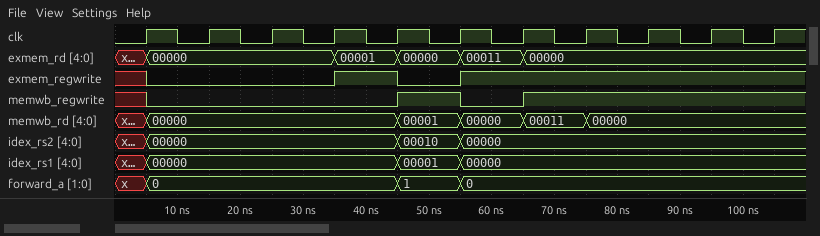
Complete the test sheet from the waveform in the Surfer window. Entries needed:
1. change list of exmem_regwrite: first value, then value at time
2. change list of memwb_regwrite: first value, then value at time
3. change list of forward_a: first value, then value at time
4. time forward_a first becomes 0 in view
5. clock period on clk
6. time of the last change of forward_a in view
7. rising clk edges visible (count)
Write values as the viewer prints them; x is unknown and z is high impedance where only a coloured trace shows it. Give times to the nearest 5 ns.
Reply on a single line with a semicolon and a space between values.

x, 0 at 5 ns, 1 at 35 ns, 0 at 45 ns, 1 at 55 ns; x, 0 at 5 ns, 1 at 45 ns, 0 at 55 ns, 1 at 65 ns; x, 0 at 5 ns, 1 at 45 ns, 0 at 55 ns; 5 ns; 10 ns; 55 ns; 11
